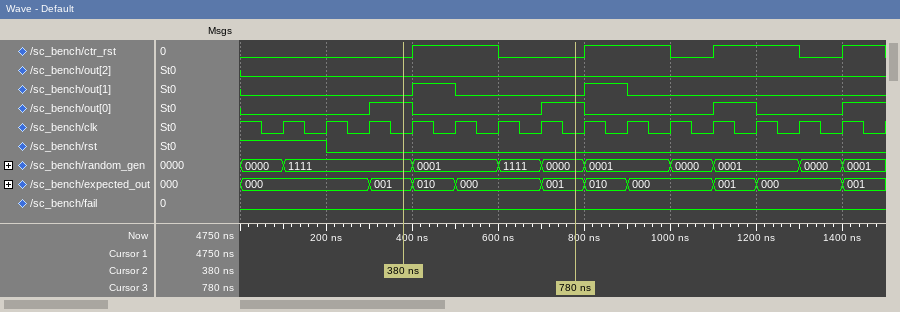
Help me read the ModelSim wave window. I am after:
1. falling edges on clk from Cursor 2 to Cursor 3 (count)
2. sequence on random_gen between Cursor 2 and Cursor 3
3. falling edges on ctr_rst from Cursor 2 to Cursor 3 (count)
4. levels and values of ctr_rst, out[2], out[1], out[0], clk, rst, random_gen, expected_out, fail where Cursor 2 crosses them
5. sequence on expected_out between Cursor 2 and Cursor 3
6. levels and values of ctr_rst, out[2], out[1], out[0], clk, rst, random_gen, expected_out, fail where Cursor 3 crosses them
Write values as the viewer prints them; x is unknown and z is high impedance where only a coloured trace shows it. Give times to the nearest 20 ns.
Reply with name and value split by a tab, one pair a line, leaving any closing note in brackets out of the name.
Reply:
falling edges on clk from Cursor 2 to Cursor 3	4
sequence on random_gen between Cursor 2 and Cursor 3	1111, 0001, 1111, 0000
falling edges on ctr_rst from Cursor 2 to Cursor 3	1
levels and values of ctr_rst, out[2], out[1], out[0], clk, rst, random_gen, expected_out, fail where Cursor 2 crosses them	ctr_rst=0, out[2]=0, out[1]=0, out[0]=1, clk=0, rst=0, random_gen=1111, expected_out=001, fail=0
sequence on expected_out between Cursor 2 and Cursor 3	001, 010, 000, 001
levels and values of ctr_rst, out[2], out[1], out[0], clk, rst, random_gen, expected_out, fail where Cursor 3 crosses them	ctr_rst=0, out[2]=0, out[1]=0, out[0]=1, clk=0, rst=0, random_gen=0000, expected_out=001, fail=0
